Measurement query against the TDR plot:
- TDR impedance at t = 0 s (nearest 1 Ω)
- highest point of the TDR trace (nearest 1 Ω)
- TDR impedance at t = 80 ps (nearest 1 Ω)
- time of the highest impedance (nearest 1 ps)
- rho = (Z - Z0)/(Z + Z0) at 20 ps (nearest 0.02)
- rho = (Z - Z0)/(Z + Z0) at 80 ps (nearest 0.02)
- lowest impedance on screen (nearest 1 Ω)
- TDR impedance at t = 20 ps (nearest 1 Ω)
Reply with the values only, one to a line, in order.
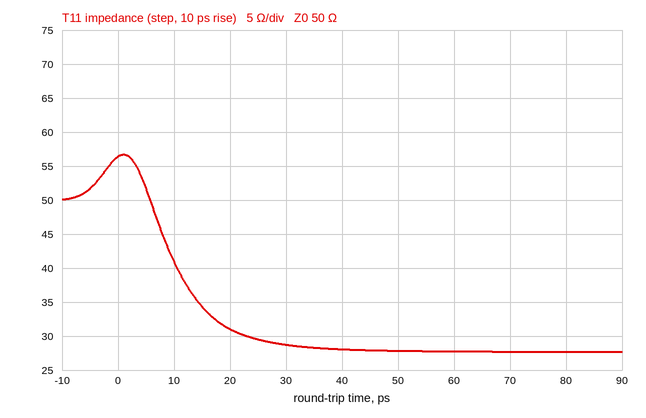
56 Ω
57 Ω
28 Ω
1 ps
-0.24
-0.28
28 Ω
31 Ω
